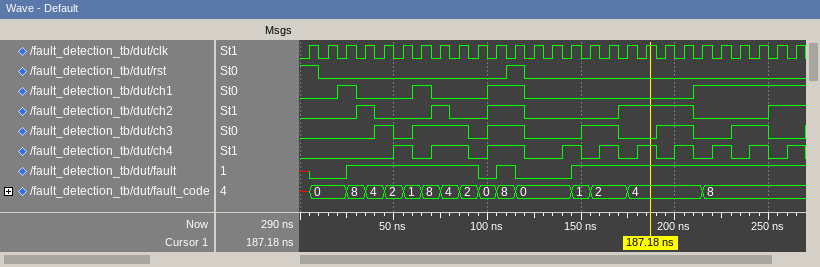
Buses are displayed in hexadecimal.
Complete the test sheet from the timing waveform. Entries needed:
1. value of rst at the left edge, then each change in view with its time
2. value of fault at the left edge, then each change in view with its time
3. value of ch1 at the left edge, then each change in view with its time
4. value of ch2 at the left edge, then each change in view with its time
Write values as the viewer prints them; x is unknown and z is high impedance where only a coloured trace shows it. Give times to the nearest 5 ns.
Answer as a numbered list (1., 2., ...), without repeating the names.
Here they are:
1. 1, 0 at 10 ns, 1 at 110 ns, 0 at 120 ns
2. x, 0 at 5 ns, 1 at 25 ns, 0 at 95 ns, 1 at 105 ns, 0 at 115 ns, 1 at 145 ns
3. 0, 1 at 20 ns, 0 at 30 ns, 1 at 60 ns, 0 at 70 ns, 1 at 100 ns, 0 at 120 ns, 1 at 210 ns
4. 0, 1 at 30 ns, 0 at 40 ns, 1 at 70 ns, 0 at 80 ns, 1 at 100 ns, 0 at 120 ns, 1 at 170 ns, 0 at 210 ns, 1 at 250 ns
